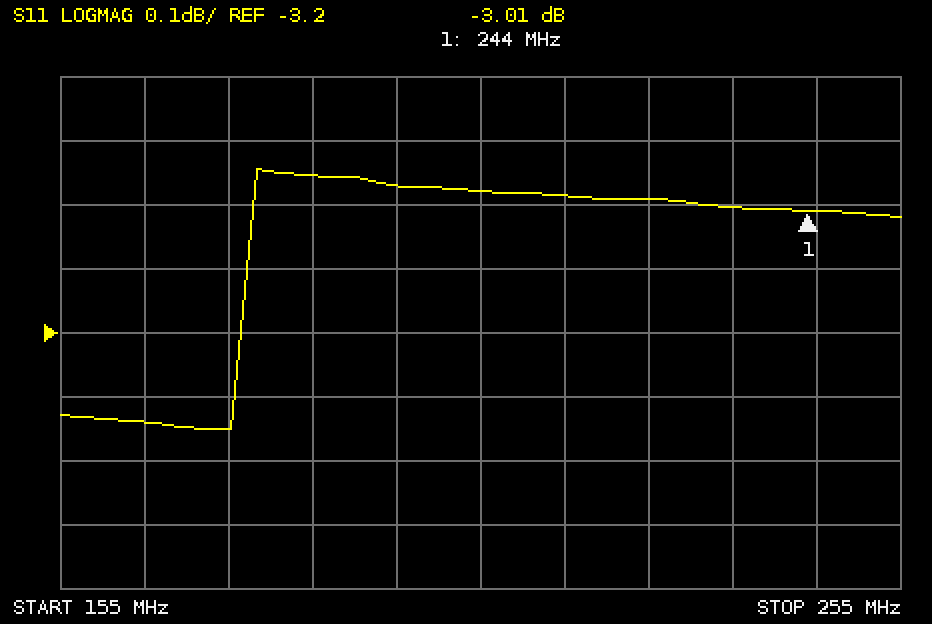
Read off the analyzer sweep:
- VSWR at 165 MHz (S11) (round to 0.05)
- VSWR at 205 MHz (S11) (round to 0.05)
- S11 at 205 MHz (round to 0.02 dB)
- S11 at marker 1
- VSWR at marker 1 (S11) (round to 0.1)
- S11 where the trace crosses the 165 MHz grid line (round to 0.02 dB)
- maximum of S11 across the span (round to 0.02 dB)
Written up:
5.25
5.90
-2.98 dB
-3.01 dB
5.8
-3.34 dB
-2.94 dB
